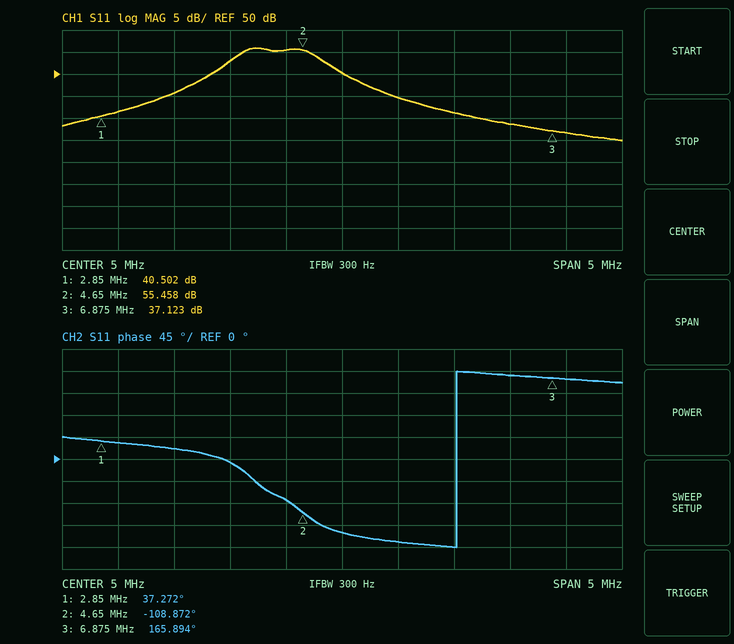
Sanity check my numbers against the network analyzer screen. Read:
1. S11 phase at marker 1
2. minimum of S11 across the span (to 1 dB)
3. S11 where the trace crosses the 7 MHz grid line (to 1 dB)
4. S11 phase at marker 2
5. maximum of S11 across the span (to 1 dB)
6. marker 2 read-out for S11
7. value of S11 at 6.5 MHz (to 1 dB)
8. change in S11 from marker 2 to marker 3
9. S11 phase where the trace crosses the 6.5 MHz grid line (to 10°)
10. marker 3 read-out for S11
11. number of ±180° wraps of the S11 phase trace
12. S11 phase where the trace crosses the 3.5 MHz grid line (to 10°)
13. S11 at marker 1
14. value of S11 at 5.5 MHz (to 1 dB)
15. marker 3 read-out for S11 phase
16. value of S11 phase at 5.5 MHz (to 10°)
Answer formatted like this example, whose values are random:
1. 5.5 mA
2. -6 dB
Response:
1. 37.272°
2. 35 dB
3. 37 dB
4. -108.872°
5. 56 dB
6. 55.458 dB
7. 39 dB
8. -18.335 dB
9. 170°
10. 37.123 dB
11. 1
12. 20°
13. 40.502 dB
14. 45 dB
15. 165.894°
16. -170°
